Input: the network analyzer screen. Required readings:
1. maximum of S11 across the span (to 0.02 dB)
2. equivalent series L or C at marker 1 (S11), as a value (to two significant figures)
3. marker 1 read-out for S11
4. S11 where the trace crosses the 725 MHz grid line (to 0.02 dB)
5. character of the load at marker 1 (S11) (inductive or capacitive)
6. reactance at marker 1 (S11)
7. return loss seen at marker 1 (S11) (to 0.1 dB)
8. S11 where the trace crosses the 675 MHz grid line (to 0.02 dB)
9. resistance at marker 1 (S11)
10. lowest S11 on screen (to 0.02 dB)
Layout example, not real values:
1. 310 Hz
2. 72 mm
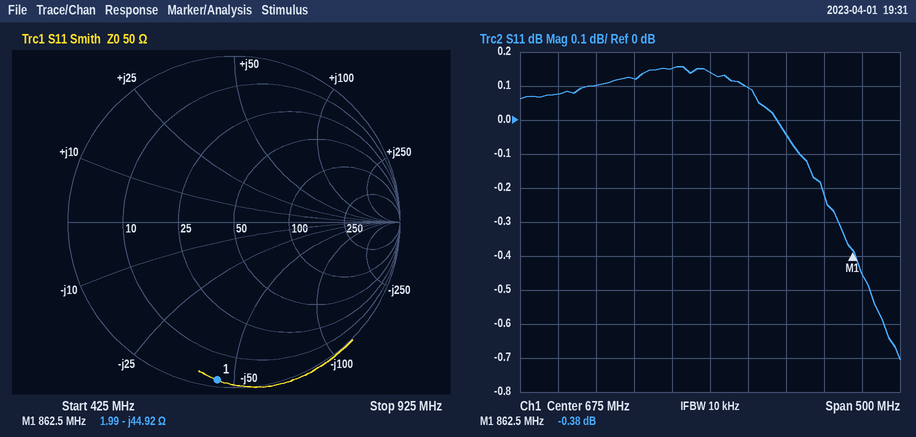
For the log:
1. 0.16 dB
2. 4.1 pF
3. -0.38 dB
4. 0.10 dB
5. capacitive
6. -44.92 Ω
7. 0.4 dB
8. 0.14 dB
9. 1.99 Ω
10. -0.70 dB
